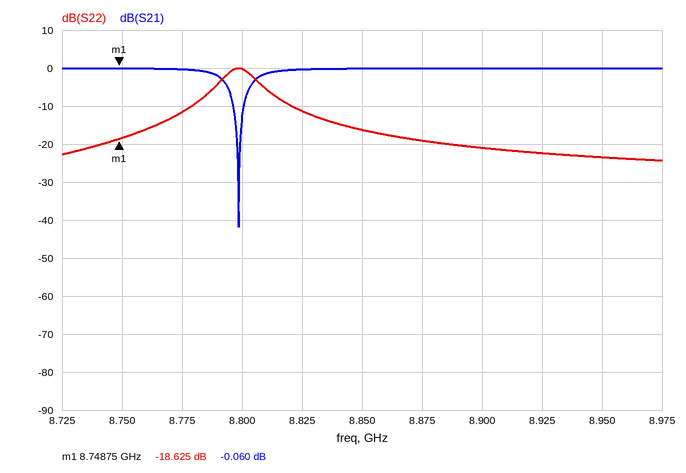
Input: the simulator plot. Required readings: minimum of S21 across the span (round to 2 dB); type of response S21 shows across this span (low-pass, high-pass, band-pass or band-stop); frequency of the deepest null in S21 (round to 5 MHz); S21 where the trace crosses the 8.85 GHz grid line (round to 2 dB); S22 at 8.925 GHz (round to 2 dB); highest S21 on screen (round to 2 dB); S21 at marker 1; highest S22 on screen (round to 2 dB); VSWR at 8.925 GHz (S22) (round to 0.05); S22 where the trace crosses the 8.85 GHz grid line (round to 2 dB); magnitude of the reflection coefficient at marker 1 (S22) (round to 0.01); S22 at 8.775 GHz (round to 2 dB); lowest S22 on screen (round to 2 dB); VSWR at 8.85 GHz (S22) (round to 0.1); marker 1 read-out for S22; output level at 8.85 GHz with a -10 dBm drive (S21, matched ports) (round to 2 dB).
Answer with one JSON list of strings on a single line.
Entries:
["-42 dB", "band-stop", "8.800 GHz", "0 dB", "-22 dB", "0 dB", "-0.060 dB", "0 dB", "1.15", "-16 dB", "0.12", "-12 dB", "-24 dB", "1.4", "-18.625 dB", "-10 dBm"]
